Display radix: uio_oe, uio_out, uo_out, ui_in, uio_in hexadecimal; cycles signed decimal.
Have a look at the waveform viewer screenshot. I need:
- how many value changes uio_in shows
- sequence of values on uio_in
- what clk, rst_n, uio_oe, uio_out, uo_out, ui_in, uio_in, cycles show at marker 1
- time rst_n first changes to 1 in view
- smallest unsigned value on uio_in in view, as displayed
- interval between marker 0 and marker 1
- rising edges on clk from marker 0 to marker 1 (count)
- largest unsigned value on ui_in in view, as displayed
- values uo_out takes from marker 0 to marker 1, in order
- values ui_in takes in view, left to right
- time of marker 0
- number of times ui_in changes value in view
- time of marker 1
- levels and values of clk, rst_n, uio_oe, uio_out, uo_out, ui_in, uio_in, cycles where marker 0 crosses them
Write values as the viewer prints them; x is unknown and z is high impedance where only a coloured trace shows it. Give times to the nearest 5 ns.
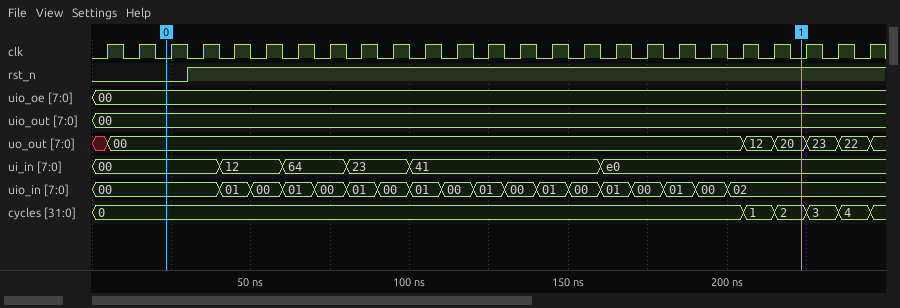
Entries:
17
00, 01, 00, 01, 00, 01, 00, 01, 00, 01, 00, 01, 00, 01, 00, 01, 00, 02
clk=0, rst_n=1, uio_oe=00, uio_out=00, uo_out=20, ui_in=e0, uio_in=02, cycles=2
30 ns
00
200 ns
20
e0
00, 12, 20
00, 12, 64, 23, 41, e0
25 ns
5
225 ns
clk=0, rst_n=0, uio_oe=00, uio_out=00, uo_out=00, ui_in=00, uio_in=00, cycles=0
